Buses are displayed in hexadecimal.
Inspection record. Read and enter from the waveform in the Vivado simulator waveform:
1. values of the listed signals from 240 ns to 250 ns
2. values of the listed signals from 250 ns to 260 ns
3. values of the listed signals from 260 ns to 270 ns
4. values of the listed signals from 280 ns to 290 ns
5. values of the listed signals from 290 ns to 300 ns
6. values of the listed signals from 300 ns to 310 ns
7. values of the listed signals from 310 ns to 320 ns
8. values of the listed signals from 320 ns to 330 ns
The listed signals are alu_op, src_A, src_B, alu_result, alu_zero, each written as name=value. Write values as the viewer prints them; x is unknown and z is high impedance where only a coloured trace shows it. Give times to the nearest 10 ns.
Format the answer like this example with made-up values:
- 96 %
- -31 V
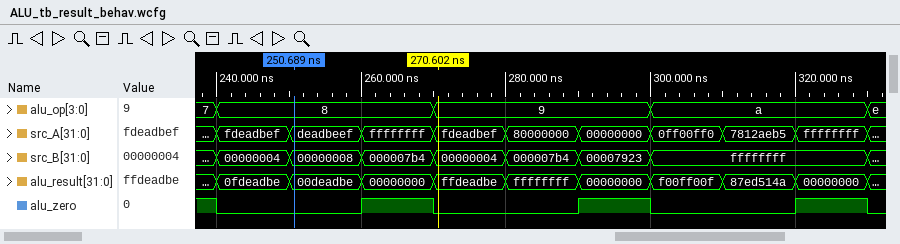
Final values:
- alu_op=8, src_A=fdeadbef, src_B=00000004, alu_result=0fdeadbe, alu_zero=0
- alu_op=8, src_A=deadbeef, src_B=00000008, alu_result=00deadbe, alu_zero=0
- alu_op=8, src_A=ffffffff, src_B=000007b4, alu_result=00000000, alu_zero=1
- alu_op=9, src_A=80000000, src_B=000007b4, alu_result=ffffffff, alu_zero=0
- alu_op=9, src_A=00000000, src_B=00007923, alu_result=00000000, alu_zero=1
- alu_op=a, src_A=0ff00ff0, src_B=ffffffff, alu_result=f00ff00f, alu_zero=0
- alu_op=a, src_A=7812aeb5, src_B=ffffffff, alu_result=87ed514a, alu_zero=0
- alu_op=a, src_A=ffffffff, src_B=ffffffff, alu_result=00000000, alu_zero=1
